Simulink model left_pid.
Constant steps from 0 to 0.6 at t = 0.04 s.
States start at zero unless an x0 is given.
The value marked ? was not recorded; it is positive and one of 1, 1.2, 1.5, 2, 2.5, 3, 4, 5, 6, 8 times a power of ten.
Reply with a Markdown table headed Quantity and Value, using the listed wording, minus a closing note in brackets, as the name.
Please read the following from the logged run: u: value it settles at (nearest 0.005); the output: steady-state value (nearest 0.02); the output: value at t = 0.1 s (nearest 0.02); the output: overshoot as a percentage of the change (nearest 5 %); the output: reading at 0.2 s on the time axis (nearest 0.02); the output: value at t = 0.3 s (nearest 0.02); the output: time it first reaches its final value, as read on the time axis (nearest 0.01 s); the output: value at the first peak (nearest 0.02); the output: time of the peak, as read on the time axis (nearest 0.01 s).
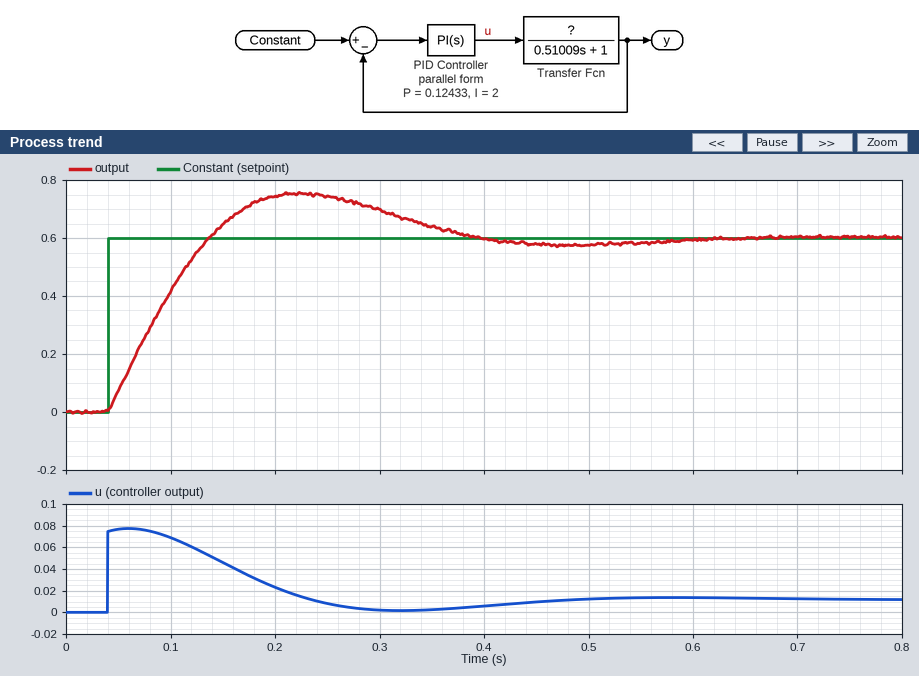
| Quantity | Value |
|---|---|
| u: value it settles at | 0.010 |
| the output: steady-state value | 0.60 |
| the output: value at t = 0.1 s | 0.42 |
| the output: overshoot as a percentage of the change | 25 % |
| the output: reading at 0.2 s on the time axis | 0.74 |
| the output: value at t = 0.3 s | 0.70 |
| the output: time it first reaches its final value, as read on the time axis | 0.14 s |
| the output: value at the first peak | 0.76 |
| the output: time of the peak, as read on the time axis | 0.22 s |
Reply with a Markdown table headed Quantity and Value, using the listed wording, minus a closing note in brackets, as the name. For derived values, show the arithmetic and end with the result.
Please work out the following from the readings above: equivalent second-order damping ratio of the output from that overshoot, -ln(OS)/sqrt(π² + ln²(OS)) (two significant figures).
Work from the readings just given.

| Quantity | Value |
|---|---|
| equivalent second-order damping ratio of the output from that overshoot, -ln(OS)/sqrt(π² + ln²(OS)) | ln(0.25) = -1.386; 1.386 / sqrt(9.870 + 1.922) = 0.40 |
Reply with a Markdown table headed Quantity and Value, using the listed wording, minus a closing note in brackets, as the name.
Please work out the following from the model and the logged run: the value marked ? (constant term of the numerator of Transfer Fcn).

| Quantity | Value |
|---|---|
| the value marked ? | 50 |
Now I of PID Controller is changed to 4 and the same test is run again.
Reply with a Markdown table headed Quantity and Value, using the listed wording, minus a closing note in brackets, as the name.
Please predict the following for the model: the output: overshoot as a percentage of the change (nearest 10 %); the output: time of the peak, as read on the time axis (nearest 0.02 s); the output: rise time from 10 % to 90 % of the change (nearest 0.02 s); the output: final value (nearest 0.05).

| Quantity | Value |
|---|---|
| the output: overshoot as a percentage of the change | 40 % |
| the output: time of the peak, as read on the time axis | 0.18 s |
| the output: rise time from 10 % to 90 % of the change | 0.06 s |
| the output: final value | 0.60 |
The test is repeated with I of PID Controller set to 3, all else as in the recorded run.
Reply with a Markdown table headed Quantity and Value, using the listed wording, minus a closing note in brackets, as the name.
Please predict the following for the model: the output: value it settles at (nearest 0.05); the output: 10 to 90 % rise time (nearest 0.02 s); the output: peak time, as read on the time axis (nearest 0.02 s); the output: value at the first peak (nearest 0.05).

| Quantity | Value |
|---|---|
| the output: value it settles at | 0.60 |
| the output: 10 to 90 % rise time | 0.06 s |
| the output: peak time, as read on the time axis | 0.20 s |
| the output: value at the first peak | 0.80 |
